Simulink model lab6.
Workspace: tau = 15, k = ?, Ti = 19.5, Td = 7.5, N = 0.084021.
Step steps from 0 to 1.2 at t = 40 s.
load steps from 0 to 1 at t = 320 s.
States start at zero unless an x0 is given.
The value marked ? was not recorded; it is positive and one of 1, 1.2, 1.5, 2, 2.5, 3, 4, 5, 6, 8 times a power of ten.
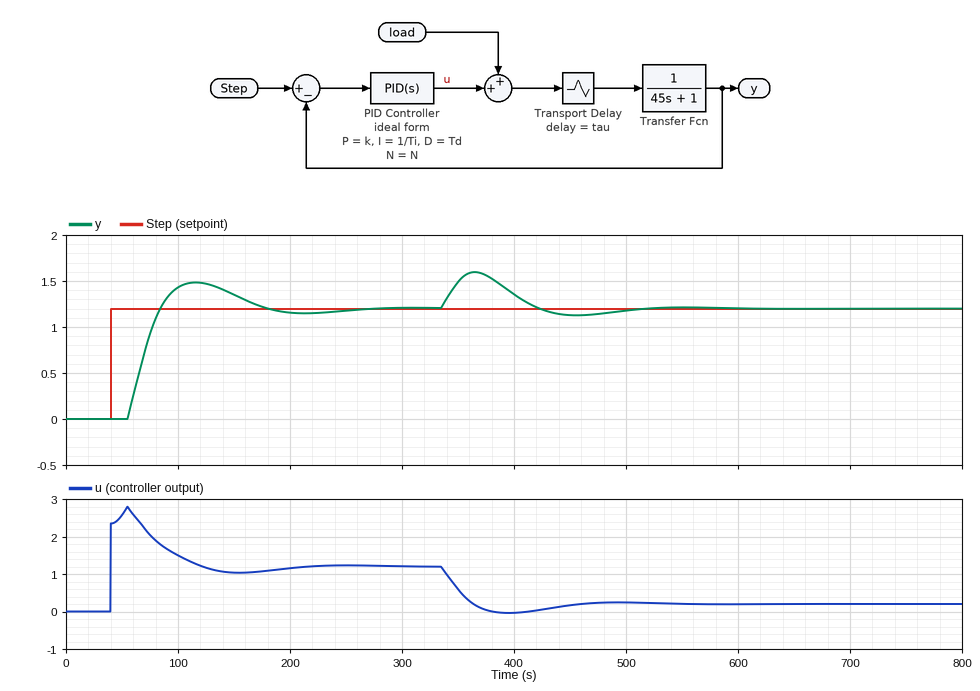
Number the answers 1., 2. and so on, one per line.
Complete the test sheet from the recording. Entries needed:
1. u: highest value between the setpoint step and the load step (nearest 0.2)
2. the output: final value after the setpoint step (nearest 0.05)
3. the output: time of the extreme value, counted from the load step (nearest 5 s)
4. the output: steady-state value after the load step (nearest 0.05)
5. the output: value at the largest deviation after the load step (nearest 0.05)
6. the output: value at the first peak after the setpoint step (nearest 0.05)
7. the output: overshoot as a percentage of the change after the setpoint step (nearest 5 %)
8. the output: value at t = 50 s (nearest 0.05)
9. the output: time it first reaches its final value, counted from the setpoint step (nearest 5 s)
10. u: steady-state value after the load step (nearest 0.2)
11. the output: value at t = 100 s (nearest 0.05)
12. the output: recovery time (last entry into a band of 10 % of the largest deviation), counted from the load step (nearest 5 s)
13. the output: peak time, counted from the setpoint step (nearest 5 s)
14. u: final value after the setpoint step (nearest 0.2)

1. 2.8
2. 1.20
3. 45 s
4. 1.20
5. 1.60
6. 1.50
7. 25 %
8. 0.00
9. 45 s
10. 0.2
11. 1.45
12. 170 s
13. 75 s
14. 1.2
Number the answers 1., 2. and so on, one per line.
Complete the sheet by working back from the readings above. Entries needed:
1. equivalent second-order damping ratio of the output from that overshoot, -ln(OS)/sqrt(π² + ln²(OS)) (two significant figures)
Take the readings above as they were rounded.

1. 0.40
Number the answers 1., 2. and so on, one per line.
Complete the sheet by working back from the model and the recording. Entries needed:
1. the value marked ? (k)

1. 1.2
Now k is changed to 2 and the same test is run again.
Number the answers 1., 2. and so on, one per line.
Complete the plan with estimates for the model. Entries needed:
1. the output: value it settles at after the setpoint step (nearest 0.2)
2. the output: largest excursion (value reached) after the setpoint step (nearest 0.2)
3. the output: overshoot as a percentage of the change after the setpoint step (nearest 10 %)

1. 1.2
2. 1.8
3. 50 %
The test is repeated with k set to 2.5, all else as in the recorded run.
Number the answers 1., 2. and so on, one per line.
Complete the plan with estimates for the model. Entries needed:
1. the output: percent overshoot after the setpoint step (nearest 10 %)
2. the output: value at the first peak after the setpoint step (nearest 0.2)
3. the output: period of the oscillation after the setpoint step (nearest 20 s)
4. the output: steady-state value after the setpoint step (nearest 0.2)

1. 70 %
2. 2.0
3. 60 s
4. 1.2
